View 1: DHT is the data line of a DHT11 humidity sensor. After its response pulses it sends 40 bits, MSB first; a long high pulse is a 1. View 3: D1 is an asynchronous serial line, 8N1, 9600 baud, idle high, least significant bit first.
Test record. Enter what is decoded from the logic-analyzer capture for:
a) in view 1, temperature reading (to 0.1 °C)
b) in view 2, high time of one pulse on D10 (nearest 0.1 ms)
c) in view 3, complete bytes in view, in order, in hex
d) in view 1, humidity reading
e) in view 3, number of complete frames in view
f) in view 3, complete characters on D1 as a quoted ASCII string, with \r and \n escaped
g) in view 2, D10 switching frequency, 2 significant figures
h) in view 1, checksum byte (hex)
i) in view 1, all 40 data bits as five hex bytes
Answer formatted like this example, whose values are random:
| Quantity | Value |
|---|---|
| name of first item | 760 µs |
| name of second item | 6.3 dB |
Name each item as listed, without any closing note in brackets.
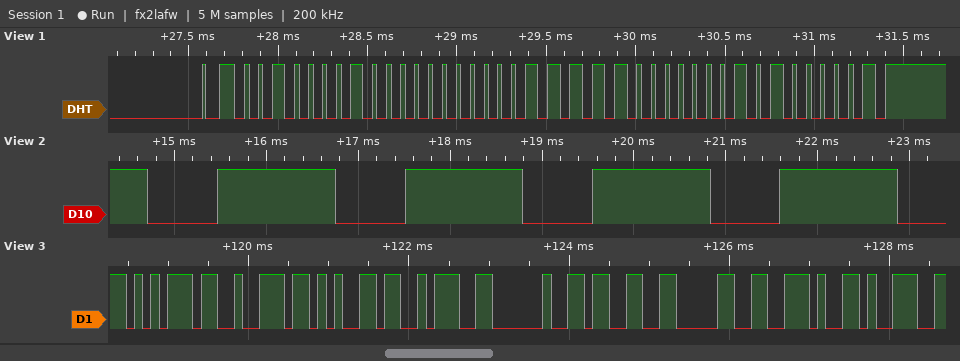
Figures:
| Quantity | Value |
|---|---|
| in view 1, temperature reading | 31.1 °C |
| in view 2, high time of one pulse on D10 | 1.3 ms |
| in view 3, complete bytes in view, in order, in hex | 75 72 65 3A 20 33 30 2E 39 |
| in view 1, humidity reading | 33 % |
| in view 3, number of complete frames in view | 9 |
| in view 3, complete characters on D1 as a quoted ASCII string, with \r and \n escaped | "ure: 30.9" |
| in view 2, D10 switching frequency, 2 significant figures | 490 Hz |
| in view 1, checksum byte | 0x41 |
| in view 1, all 40 data bits as five hex bytes | 21 00 1F 01 41 |
